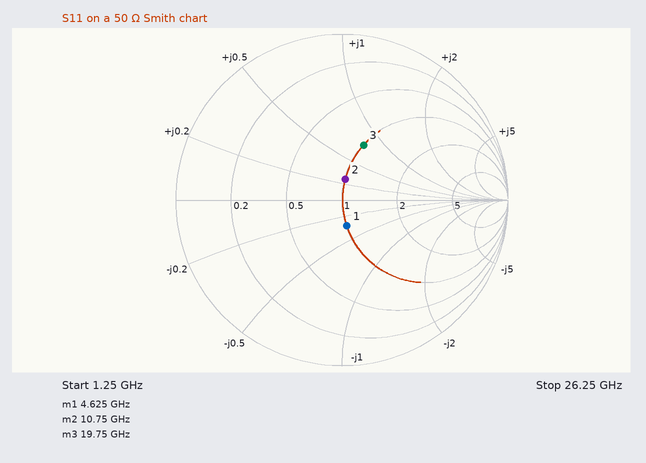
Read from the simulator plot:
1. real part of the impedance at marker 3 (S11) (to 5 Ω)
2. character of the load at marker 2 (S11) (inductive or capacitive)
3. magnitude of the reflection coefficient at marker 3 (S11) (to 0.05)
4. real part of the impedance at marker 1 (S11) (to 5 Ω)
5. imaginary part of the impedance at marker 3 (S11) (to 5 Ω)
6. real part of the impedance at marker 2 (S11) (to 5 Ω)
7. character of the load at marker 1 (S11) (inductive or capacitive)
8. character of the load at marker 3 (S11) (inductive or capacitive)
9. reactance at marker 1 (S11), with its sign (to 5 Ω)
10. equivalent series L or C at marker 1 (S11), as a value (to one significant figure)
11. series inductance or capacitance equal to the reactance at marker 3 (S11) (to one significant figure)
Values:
50 Ω
inductive
0.35
50 Ω
+40 Ω
50 Ω
capacitive
inductive
-15 Ω
2 pF
300 pH
